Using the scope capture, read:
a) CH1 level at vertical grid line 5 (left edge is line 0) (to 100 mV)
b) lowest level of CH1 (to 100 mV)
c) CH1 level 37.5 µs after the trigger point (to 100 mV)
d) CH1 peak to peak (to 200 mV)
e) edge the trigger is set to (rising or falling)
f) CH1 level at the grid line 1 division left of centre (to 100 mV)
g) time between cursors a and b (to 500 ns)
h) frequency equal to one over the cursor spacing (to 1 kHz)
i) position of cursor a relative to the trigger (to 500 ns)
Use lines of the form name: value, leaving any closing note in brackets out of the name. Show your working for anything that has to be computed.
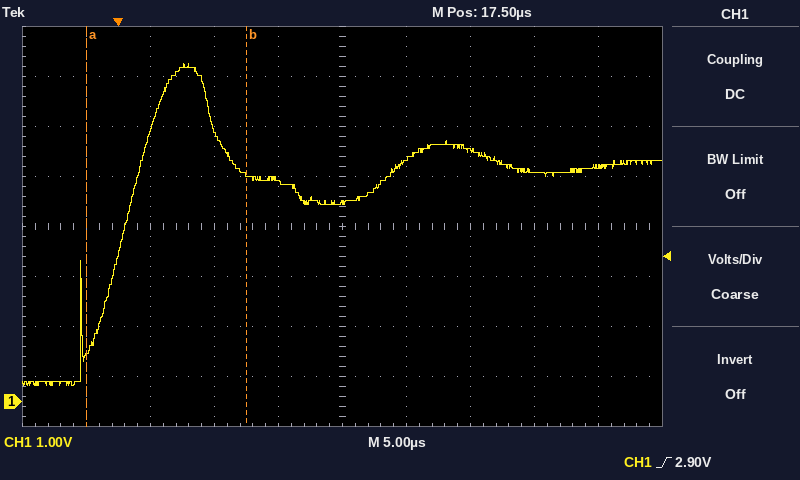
CH1 level at vertical grid line 5 (left edge is line 0): 4.0 V
lowest level of CH1: 300 mV
CH1 level 37.5 µs after the trigger point: 4.7 V
CH1 peak to peak: 6.4 V
edge the trigger is set to: rising
CH1 level at the grid line 1 division left of centre: 4.4 V
time between cursors a and b: 12.5 µs
frequency equal to one over the cursor spacing: 1 / 12.5 µs ≈ 80 kHz
position of cursor a relative to the trigger: -2.5 µs
